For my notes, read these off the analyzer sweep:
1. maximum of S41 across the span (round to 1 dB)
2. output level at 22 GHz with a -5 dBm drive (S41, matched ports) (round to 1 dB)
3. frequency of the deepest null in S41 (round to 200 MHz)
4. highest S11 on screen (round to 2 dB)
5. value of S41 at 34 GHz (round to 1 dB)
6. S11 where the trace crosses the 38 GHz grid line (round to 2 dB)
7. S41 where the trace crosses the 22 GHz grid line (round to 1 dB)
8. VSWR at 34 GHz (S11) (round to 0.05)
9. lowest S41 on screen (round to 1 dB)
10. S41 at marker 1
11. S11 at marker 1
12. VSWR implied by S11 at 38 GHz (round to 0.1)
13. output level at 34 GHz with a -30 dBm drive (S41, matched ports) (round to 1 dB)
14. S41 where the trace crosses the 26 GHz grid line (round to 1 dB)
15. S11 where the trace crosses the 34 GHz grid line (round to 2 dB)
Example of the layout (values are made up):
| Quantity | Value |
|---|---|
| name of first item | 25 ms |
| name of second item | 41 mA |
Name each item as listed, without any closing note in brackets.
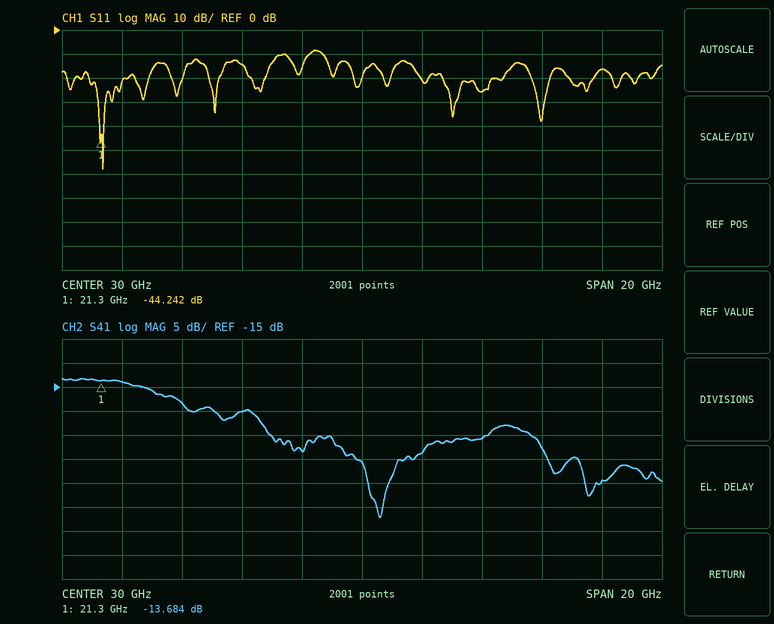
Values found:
| Quantity | Value |
|---|---|
| maximum of S41 across the span | -13 dB |
| output level at 22 GHz with a -5 dBm drive (S41, matched ports) | -19 dBm |
| frequency of the deepest null in S41 | 30.6 GHz |
| highest S11 on screen | -8 dB |
| value of S41 at 34 GHz | -26 dB |
| S11 where the trace crosses the 38 GHz grid line | -16 dB |
| S41 where the trace crosses the 22 GHz grid line | -14 dB |
| VSWR at 34 GHz (S11) | 1.10 |
| lowest S41 on screen | -42 dB |
| S41 at marker 1 | -13.684 dB |
| S11 at marker 1 | -44.242 dB |
| VSWR implied by S11 at 38 GHz | 1.4 |
| output level at 34 GHz with a -30 dBm drive (S41, matched ports) | -56 dBm |
| S41 where the trace crosses the 26 GHz grid line | -20 dB |
| S11 where the trace crosses the 34 GHz grid line | -26 dB |
